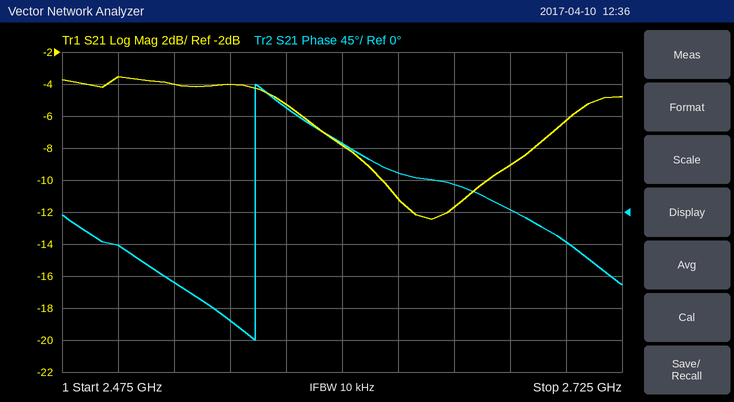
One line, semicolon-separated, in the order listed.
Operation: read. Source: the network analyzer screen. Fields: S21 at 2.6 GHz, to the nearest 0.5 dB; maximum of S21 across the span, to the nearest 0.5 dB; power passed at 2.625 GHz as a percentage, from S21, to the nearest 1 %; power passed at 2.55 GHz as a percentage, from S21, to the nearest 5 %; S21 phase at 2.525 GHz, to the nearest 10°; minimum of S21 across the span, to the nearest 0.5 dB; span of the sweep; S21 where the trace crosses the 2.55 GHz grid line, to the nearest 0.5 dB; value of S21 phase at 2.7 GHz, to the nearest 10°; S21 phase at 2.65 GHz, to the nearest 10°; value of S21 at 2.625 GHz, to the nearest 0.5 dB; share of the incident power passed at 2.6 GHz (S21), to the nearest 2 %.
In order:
-8.0 dB; -3.5 dB; 8 %; 40 %; -100°; -12.5 dB; 250 MHz; -4.0 dB; -40°; 40°; -11.0 dB; 16 %
